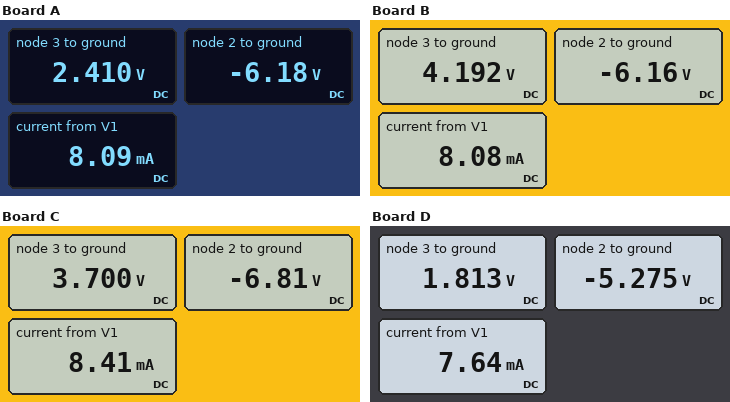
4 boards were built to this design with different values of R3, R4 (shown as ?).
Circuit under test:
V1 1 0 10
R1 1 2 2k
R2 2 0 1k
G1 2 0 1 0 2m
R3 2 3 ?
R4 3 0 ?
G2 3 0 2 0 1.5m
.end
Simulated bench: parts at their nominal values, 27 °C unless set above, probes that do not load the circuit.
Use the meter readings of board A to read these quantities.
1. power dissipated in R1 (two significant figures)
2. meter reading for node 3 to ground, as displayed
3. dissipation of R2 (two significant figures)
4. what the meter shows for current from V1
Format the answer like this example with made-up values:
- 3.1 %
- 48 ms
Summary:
- 130 mW
- 2.410 V
- 38 mW
- 8.09 mA
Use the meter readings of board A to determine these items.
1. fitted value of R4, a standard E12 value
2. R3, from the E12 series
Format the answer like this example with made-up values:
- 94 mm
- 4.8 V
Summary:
- 680 Ω
- 1.5 kΩ
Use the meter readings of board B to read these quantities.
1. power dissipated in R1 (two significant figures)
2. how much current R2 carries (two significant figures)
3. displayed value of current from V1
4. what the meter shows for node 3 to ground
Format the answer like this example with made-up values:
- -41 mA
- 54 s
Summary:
- 130 mW
- 6.2 mA
- 8.08 mA
- 4.192 V
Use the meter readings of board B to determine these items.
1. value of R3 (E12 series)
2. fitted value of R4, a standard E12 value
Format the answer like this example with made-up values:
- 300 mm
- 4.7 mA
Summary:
- 1.8 kΩ
- 1.2 kΩ
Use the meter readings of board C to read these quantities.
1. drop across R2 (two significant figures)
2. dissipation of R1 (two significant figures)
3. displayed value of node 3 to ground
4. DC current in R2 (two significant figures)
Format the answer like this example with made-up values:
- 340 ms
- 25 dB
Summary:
- 6.8 V
- 140 mW
- 3.700 V
- 6.8 mA
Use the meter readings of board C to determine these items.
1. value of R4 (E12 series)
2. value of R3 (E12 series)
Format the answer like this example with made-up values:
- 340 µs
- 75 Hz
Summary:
- 680 Ω
- 2.2 kΩ
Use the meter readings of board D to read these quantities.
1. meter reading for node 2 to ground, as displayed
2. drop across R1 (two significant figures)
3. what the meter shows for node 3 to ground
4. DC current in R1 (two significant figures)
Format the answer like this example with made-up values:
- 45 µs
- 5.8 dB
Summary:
- -5.275 V
- 15 V
- 1.813 V
- 7.6 mA
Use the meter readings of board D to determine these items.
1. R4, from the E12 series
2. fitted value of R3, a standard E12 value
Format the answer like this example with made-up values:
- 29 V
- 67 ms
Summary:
- 2.2 kΩ
- 1 kΩ
